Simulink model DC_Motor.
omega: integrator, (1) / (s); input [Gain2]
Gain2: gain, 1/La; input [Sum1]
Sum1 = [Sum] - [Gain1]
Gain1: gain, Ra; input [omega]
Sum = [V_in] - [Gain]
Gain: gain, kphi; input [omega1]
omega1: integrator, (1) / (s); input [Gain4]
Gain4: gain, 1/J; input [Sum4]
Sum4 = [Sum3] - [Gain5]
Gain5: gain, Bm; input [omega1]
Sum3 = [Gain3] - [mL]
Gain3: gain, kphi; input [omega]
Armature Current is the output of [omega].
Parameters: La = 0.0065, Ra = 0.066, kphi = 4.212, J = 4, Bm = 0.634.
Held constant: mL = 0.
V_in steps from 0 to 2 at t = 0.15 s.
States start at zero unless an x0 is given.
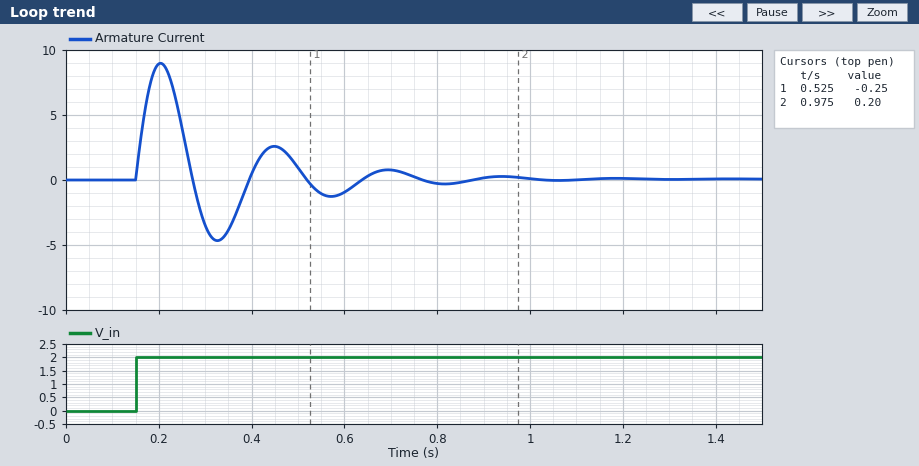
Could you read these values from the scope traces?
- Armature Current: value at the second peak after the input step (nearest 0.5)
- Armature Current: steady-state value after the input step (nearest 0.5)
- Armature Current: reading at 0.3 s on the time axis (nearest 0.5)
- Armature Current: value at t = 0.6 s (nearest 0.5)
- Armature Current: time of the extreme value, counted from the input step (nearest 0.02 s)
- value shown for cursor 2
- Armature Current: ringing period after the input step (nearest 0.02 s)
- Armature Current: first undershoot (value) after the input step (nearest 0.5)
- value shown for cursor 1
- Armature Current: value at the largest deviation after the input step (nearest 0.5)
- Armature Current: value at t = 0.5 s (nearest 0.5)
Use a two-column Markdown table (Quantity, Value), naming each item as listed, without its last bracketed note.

| Quantity | Value |
|---|---|
| Armature Current: value at the second peak after the input step | 2.5 |
| Armature Current: steady-state value after the input step | 0.0 |
| Armature Current: reading at 0.3 s on the time axis | -3.5 |
| Armature Current: value at t = 0.6 s | -1.0 |
| Armature Current: time of the extreme value, counted from the input step | 0.06 s |
| value shown for cursor 2 | 0.20 |
| Armature Current: ringing period after the input step | 0.24 s |
| Armature Current: first undershoot (value) after the input step | -4.5 |
| value shown for cursor 1 | -0.25 |
| Armature Current: value at the largest deviation after the input step | 9.0 |
| Armature Current: value at t = 0.5 s | 1.0 |
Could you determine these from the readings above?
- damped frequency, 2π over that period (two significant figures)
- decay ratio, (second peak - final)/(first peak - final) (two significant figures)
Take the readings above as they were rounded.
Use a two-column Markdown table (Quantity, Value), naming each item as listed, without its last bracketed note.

| Quantity | Value |
|---|---|
| damped frequency, 2π over that period | 26 rad/s |
| decay ratio, (second peak - final)/(first peak - final) | 0.28 |
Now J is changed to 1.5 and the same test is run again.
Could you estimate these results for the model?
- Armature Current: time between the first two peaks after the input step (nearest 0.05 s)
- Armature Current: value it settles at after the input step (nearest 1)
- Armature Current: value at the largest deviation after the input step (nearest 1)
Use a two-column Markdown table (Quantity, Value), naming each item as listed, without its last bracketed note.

| Quantity | Value |
|---|---|
| Armature Current: time between the first two peaks after the input step | 0.15 s |
| Armature Current: value it settles at after the input step | 0 |
| Armature Current: value at the largest deviation after the input step | 6 |
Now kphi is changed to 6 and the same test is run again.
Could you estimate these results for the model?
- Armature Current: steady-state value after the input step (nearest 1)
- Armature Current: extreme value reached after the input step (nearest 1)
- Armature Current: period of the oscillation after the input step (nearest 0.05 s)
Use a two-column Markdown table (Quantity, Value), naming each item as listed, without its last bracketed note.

| Quantity | Value |
|---|---|
| Armature Current: steady-state value after the input step | 0 |
| Armature Current: extreme value reached after the input step | 7 |
| Armature Current: period of the oscillation after the input step | 0.15 s |
